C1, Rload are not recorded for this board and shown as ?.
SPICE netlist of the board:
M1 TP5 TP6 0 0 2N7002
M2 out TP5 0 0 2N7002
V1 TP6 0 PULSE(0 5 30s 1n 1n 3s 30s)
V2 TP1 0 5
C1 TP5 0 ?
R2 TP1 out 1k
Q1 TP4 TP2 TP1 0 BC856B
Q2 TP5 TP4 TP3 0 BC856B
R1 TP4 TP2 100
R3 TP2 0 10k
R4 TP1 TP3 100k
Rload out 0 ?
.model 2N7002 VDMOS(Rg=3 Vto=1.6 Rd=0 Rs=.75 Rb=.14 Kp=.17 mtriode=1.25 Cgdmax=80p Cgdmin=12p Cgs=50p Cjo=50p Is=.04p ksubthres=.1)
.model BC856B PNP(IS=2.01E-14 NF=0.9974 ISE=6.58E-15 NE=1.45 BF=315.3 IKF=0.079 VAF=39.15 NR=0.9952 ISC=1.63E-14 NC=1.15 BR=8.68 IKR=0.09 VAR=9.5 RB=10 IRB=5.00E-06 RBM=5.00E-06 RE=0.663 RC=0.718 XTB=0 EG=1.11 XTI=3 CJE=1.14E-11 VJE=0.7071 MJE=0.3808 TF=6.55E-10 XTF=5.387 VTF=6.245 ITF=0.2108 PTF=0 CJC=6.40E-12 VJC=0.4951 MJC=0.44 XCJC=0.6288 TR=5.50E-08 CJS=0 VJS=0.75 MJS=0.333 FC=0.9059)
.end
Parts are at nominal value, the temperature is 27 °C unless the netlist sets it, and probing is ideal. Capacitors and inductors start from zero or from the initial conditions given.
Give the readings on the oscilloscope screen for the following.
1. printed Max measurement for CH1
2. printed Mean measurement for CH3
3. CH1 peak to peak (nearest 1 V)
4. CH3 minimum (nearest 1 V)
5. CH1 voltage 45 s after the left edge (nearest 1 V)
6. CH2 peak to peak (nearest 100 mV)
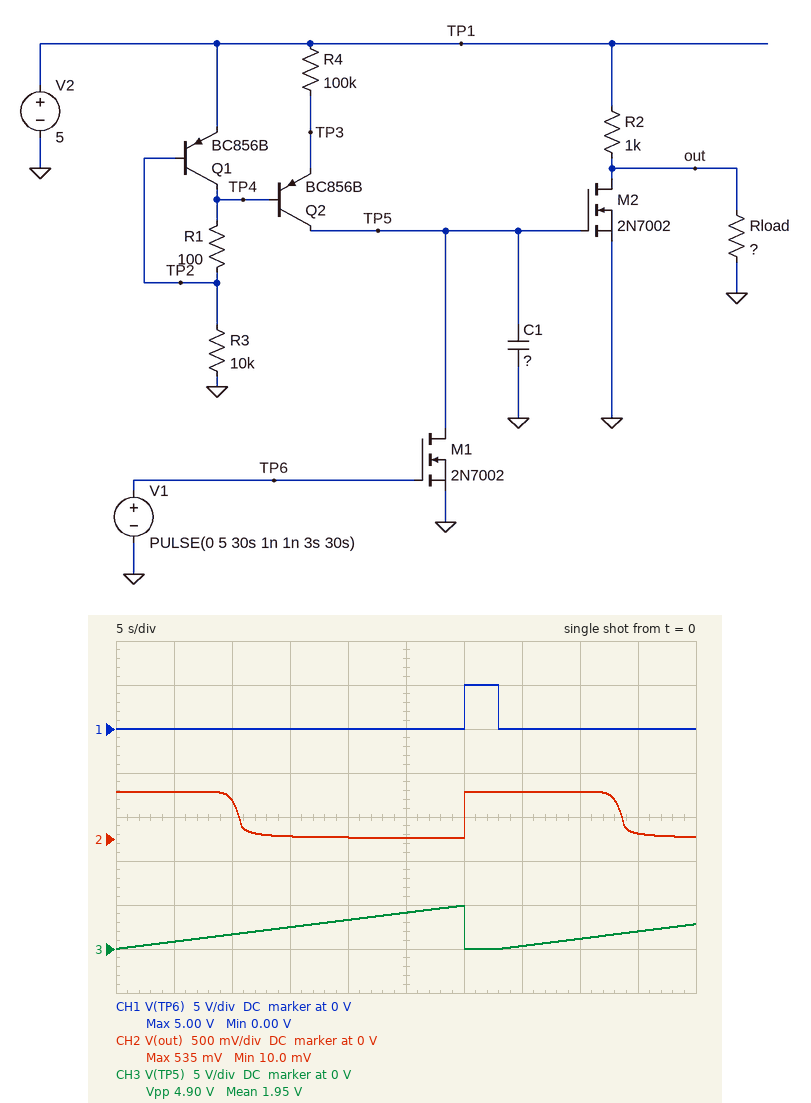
5.00 V
1.95 V
5 V
0 V
0 V
500 mV
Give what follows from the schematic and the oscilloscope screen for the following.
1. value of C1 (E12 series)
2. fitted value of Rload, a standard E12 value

6.8 µF
120 Ω
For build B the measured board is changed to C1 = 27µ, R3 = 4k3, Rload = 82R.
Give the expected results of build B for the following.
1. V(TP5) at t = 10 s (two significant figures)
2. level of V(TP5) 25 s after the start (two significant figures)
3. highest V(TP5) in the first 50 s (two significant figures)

320 mV
790 mV
950 mV
